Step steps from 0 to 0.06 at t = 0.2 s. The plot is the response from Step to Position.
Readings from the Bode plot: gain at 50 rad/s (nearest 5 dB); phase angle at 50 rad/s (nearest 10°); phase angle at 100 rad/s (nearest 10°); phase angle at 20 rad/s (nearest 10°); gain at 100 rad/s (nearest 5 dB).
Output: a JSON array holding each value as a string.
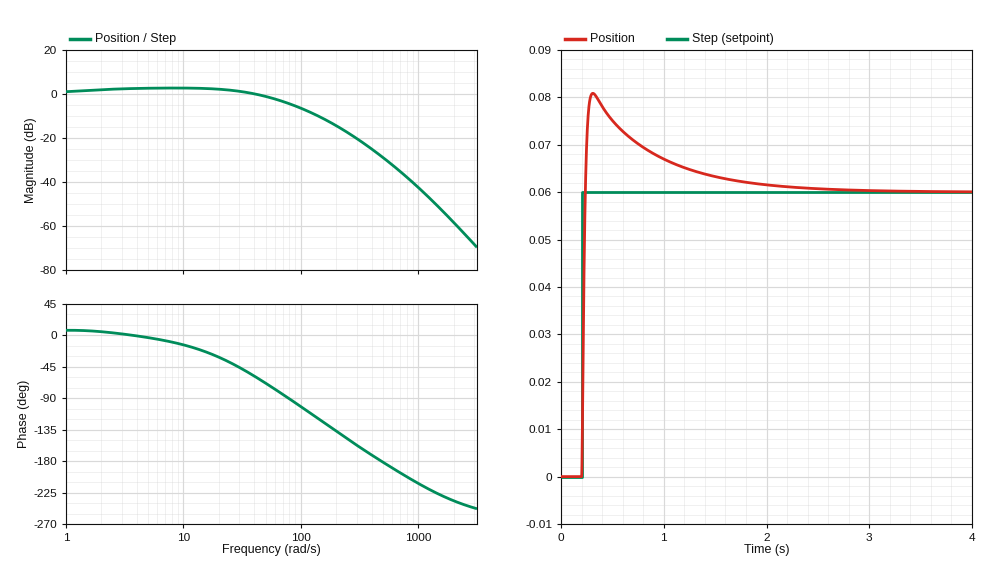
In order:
["0 dB", "-70°", "-100°", "-30°", "-5 dB"]
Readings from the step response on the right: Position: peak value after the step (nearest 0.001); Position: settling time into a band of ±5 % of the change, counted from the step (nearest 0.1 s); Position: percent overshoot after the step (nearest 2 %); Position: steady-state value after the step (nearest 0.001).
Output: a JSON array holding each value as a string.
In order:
["0.081", "1.4 s", "34 %", "0.060"]
